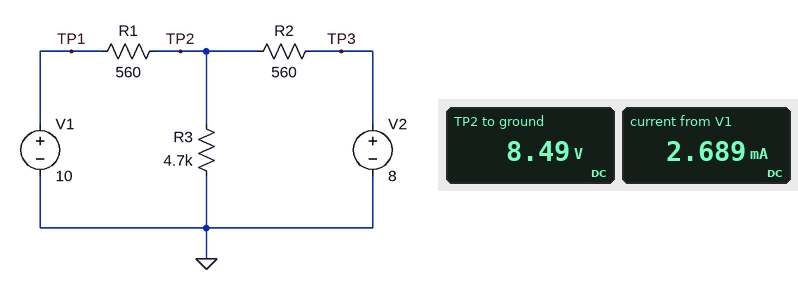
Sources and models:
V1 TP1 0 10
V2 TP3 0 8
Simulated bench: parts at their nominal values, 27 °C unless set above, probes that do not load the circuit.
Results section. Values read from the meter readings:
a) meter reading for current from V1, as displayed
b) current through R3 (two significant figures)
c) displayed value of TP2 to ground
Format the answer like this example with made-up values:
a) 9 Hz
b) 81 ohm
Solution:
a) 2.689 mA
b) 1.8 mA
c) 8.49 V
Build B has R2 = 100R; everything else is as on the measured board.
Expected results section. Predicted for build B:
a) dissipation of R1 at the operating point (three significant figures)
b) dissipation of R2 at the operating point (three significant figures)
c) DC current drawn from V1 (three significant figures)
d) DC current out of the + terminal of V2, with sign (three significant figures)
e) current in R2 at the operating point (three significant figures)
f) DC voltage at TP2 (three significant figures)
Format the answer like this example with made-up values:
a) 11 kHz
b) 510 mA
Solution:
a) 6.07 mW
b) 243 µW
c) 3.29 mA
d) -1.56 mA
e) 1.56 mA
f) 8.16 V
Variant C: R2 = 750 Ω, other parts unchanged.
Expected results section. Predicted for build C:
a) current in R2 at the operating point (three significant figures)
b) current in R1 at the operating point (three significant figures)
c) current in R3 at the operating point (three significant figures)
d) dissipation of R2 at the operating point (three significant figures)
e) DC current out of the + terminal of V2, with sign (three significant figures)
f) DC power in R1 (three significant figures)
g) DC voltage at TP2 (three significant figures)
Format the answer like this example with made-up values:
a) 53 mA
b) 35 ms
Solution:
a) 748 µA
b) 2.57 mA
c) 1.82 mA
d) 420 µW
e) -748 µA
f) 3.70 mW
g) 8.56 V
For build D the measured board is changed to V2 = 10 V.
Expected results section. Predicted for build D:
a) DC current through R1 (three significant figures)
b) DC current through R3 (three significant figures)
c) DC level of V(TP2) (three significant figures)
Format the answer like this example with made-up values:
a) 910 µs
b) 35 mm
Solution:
a) 1.00 mA
b) 2.01 mA
c) 9.44 V
